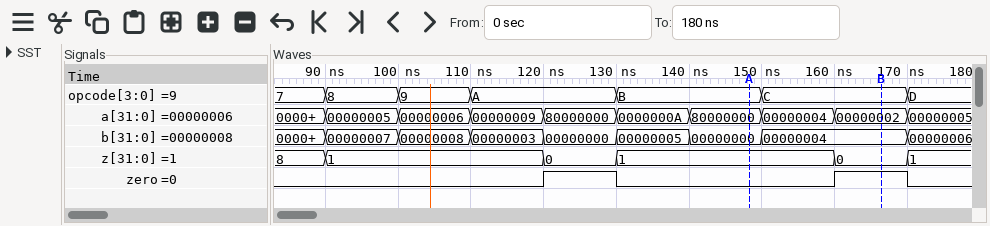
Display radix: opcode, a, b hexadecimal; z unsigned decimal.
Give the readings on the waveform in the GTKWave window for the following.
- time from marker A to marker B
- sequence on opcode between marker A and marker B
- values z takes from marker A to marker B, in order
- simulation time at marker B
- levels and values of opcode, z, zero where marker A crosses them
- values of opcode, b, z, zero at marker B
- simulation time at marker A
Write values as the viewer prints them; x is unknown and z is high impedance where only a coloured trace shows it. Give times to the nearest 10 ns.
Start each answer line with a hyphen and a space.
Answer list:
- 20 ns
- B, C
- 1, 0
- 170 ns
- opcode=B, z=1, zero=0
- opcode=C, b=00000004, z=0, zero=1
- 150 ns
